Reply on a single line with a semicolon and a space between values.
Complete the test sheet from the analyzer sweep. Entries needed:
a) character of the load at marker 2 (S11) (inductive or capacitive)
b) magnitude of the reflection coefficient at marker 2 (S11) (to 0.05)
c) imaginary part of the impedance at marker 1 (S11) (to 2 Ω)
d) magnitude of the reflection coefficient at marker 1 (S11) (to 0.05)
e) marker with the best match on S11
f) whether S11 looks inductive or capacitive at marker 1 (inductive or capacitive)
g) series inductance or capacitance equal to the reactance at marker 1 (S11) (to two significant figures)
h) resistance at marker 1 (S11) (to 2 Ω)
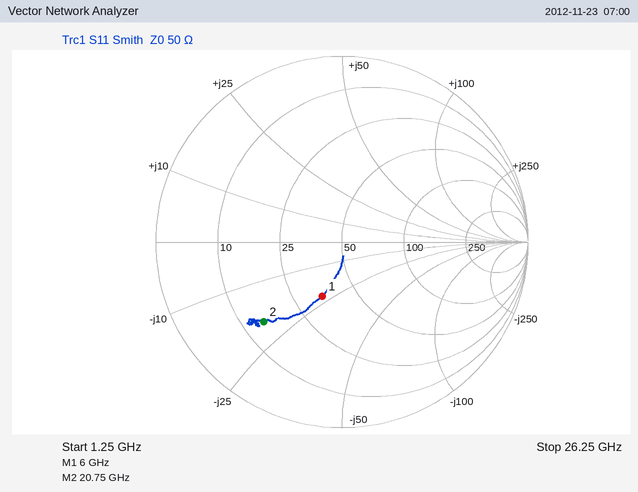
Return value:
capacitive; 0.60; -22 Ω; 0.30; marker 1; capacitive; 1.2 pF; 34 Ω
